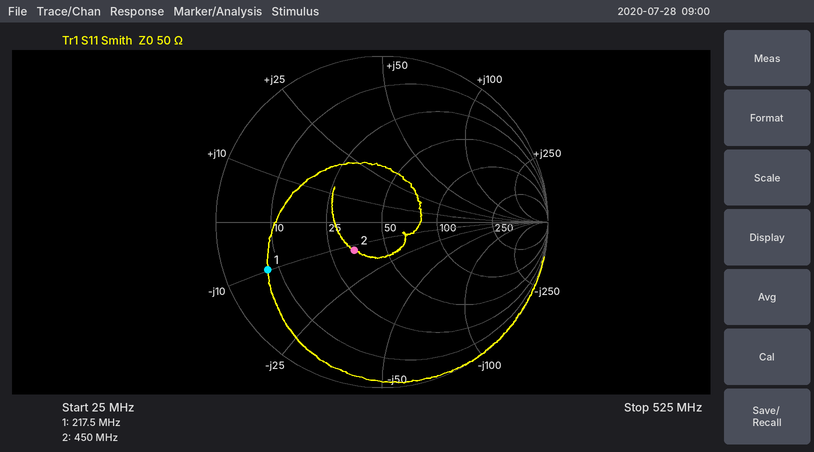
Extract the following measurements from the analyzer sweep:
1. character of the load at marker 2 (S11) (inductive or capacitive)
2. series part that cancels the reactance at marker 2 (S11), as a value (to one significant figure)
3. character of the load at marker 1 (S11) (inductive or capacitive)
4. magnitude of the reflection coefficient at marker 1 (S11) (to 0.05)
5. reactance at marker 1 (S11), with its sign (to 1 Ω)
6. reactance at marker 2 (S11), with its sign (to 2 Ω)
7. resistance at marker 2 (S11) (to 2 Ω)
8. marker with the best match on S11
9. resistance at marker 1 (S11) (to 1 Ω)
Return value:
capacitive
4 nH
capacitive
0.75
-10 Ω
-12 Ω
34 Ω
marker 2
8 Ω
